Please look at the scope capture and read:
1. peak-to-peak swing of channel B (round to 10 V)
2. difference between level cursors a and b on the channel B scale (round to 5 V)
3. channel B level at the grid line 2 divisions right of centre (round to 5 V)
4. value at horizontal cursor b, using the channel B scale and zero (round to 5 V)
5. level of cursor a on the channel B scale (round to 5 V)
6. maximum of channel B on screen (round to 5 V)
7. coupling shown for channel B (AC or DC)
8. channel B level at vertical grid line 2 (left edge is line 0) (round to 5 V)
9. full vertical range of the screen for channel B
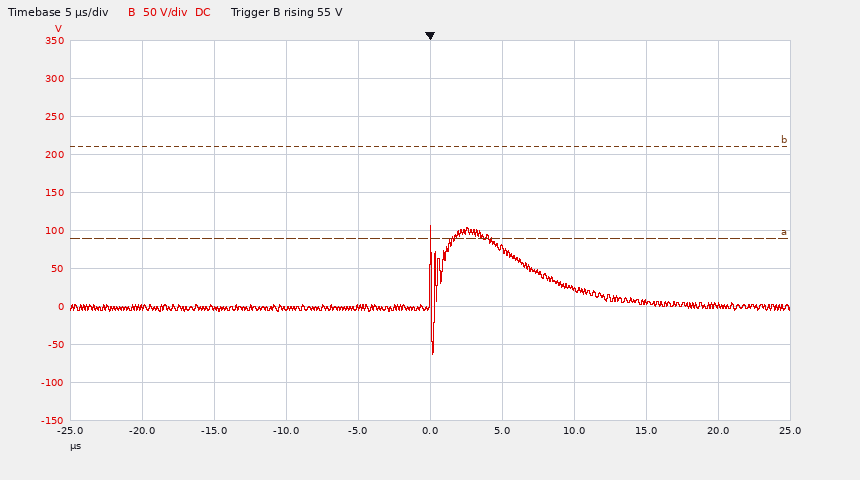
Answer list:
170 V
120 V
25 V
210 V
90 V
105 V
DC
0 V
500 V
